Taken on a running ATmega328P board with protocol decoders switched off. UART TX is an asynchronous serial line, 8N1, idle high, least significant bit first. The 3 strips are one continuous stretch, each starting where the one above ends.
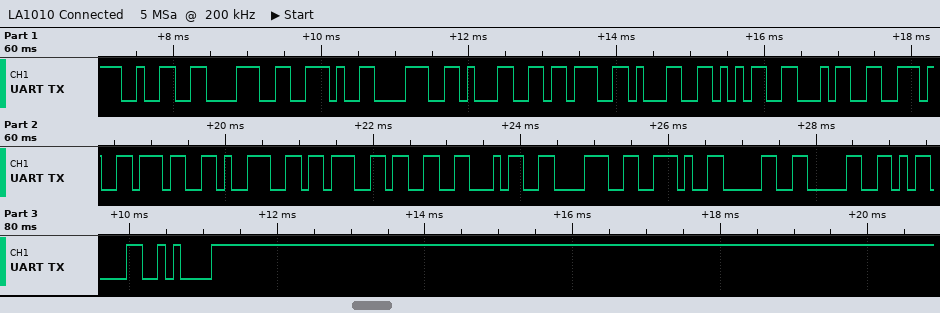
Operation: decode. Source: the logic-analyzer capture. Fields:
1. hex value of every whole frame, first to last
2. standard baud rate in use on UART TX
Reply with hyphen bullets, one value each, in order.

- 32 38 2E 38 31 3B 31 35 34 2E 37 39 3B 33 34 38 2E 30 30 0D 0A
- 9600 baud
